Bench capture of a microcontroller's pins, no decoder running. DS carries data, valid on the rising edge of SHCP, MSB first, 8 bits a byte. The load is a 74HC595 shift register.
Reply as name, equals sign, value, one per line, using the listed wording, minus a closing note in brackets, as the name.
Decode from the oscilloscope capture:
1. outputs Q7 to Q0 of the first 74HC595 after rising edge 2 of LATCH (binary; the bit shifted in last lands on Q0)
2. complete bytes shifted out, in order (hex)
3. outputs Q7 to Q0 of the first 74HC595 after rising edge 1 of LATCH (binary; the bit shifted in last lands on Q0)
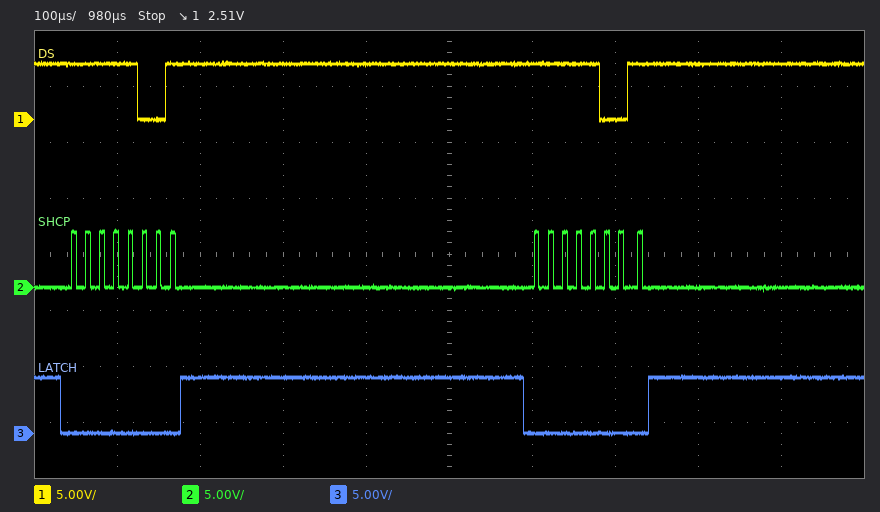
outputs Q7 to Q0 of the first 74HC595 after rising edge 2 of LATCH = 11111001
complete bytes shifted out, in order = F9 F9
outputs Q7 to Q0 of the first 74HC595 after rising edge 1 of LATCH = 11111001
